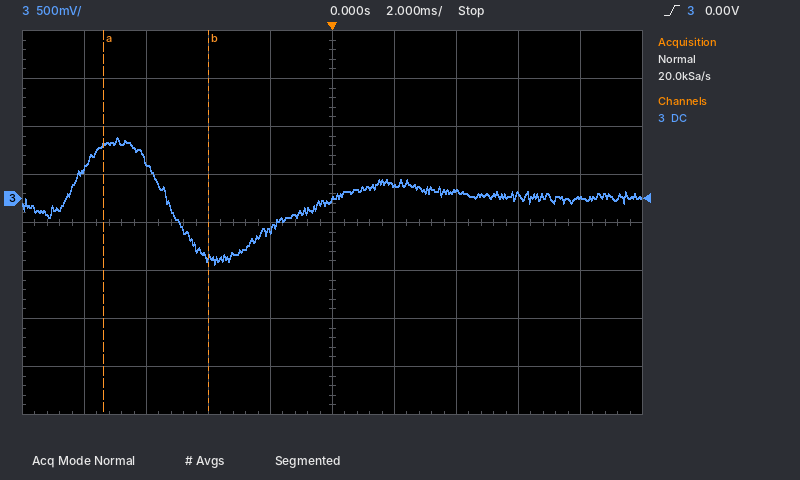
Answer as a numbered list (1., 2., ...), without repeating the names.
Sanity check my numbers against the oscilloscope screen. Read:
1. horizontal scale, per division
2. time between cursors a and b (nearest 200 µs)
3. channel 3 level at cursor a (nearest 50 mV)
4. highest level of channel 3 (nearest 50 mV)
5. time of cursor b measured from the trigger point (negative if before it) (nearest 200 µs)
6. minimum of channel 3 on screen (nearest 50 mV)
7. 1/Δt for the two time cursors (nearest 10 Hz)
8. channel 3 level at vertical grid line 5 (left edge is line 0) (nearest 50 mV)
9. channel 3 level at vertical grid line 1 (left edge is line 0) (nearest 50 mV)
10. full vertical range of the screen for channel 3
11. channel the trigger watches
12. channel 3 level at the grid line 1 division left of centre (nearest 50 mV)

1. 2 ms
2. 3.4 ms
3. 550 mV
4. 650 mV
5. -4.0 ms
6. -700 mV
7. 290 Hz
8. 0 mV
9. 300 mV
10. 4 V
11. channel 3
12. -300 mV
